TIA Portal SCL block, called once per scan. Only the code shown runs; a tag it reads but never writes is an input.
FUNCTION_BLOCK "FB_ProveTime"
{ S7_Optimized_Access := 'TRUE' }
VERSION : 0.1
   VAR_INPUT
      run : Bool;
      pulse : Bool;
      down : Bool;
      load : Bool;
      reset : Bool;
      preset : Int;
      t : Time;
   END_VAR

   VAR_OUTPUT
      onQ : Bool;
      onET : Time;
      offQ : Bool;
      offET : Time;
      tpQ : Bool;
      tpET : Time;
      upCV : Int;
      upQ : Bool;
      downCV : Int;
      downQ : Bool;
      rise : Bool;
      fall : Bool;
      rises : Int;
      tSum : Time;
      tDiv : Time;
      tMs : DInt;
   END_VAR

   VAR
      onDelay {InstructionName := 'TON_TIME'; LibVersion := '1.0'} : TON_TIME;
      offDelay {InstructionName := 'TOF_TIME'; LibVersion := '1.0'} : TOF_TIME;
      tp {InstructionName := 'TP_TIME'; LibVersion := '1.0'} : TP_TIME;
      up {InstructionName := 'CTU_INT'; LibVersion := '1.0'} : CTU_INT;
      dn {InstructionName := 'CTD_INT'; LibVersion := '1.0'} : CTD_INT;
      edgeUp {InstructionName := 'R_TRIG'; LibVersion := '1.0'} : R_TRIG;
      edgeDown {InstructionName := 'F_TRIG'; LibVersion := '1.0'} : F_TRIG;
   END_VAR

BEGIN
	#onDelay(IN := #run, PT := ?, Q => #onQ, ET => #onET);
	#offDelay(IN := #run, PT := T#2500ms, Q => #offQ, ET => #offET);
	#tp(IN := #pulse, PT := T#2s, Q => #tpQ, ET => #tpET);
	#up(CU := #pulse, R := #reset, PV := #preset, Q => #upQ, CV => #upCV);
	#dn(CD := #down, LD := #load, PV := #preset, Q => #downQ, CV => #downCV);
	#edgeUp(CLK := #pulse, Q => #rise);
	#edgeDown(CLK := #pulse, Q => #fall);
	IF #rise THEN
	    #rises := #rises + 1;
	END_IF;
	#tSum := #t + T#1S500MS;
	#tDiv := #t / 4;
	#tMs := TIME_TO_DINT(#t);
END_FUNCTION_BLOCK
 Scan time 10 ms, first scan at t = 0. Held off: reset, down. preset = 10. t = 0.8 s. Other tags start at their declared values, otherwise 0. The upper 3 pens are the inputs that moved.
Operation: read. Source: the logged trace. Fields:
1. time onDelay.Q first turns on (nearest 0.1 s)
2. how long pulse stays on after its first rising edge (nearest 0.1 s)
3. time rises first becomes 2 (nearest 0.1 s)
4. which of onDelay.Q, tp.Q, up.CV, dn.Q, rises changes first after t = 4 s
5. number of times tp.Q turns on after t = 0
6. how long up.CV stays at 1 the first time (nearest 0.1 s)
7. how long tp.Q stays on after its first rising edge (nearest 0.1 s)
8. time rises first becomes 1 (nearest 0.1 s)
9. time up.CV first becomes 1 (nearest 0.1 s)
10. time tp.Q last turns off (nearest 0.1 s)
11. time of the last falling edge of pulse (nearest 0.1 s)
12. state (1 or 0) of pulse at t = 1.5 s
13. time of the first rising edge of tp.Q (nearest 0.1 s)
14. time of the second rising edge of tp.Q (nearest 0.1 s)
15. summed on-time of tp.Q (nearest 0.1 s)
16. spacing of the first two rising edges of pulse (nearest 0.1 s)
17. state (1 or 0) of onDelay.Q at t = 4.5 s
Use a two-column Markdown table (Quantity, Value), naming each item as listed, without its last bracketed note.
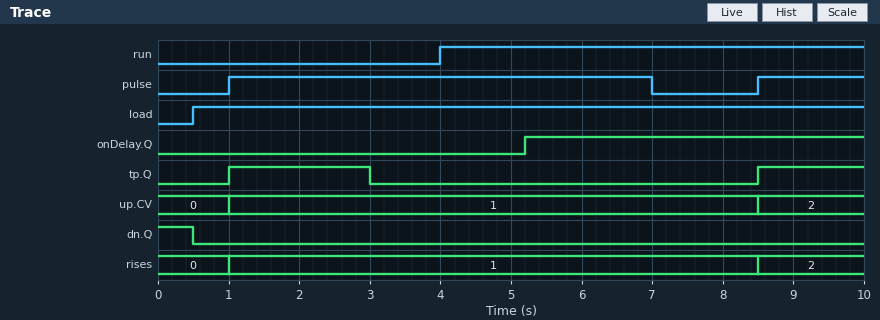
| Quantity | Value |
|---|---|
| time onDelay.Q first turns on | 5.2 s |
| how long pulse stays on after its first rising edge | 6.0 s |
| time rises first becomes 2 | 8.5 s |
| which of onDelay.Q, tp.Q, up.CV, dn.Q, rises changes first after t = 4 s | onDelay.Q |
| number of times tp.Q turns on after t = 0 | 2 |
| how long up.CV stays at 1 the first time | 7.5 s |
| how long tp.Q stays on after its first rising edge | 2.0 s |
| time rises first becomes 1 | 1.0 s |
| time up.CV first becomes 1 | 1.0 s |
| time tp.Q last turns off | 3.0 s |
| time of the last falling edge of pulse | 7.0 s |
| state (1 or 0) of pulse at t = 1.5 s | 1 |
| time of the first rising edge of tp.Q | 1.0 s |
| time of the second rising edge of tp.Q | 8.5 s |
| summed on-time of tp.Q | 3.5 s |
| spacing of the first two rising edges of pulse | 7.5 s |
| state (1 or 0) of onDelay.Q at t = 4.5 s | 0 |
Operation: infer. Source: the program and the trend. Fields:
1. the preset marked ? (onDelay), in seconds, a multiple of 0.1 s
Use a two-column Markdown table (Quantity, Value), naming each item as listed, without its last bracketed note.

| Quantity | Value |
|---|---|
| the preset marked ? (onDelay), in seconds, a multiple of 0.1 s | 1.2 s |
